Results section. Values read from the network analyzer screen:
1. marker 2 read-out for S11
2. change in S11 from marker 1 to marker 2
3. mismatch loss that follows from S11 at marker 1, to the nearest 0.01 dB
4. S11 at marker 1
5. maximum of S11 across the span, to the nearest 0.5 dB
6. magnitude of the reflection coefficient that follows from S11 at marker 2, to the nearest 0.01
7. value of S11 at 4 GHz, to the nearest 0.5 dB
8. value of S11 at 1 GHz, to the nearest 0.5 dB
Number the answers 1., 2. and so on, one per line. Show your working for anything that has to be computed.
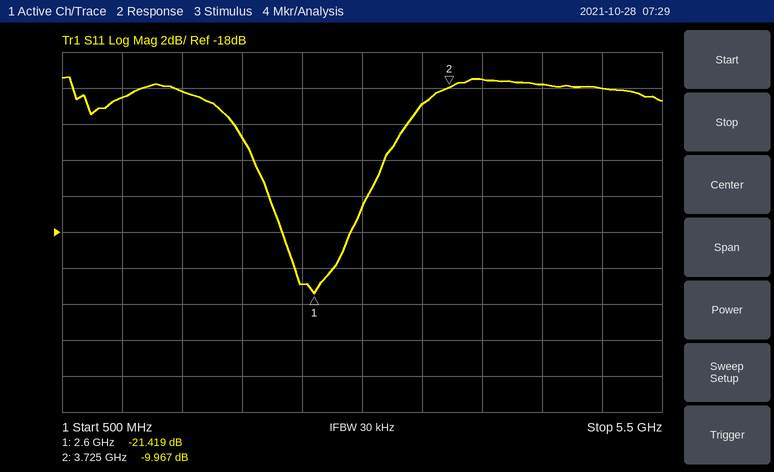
1. -9.967 dB
2. -9.967 − (-21.419) = 11.452 dB
3. −10 log10(1 − 10^(-21.419/10)) ≈ 0.03 dB
4. -21.419 dB
5. -9.5 dB
6. 10^(-9.967/20) ≈ 0.32
7. -9.5 dB
8. -10.5 dB
